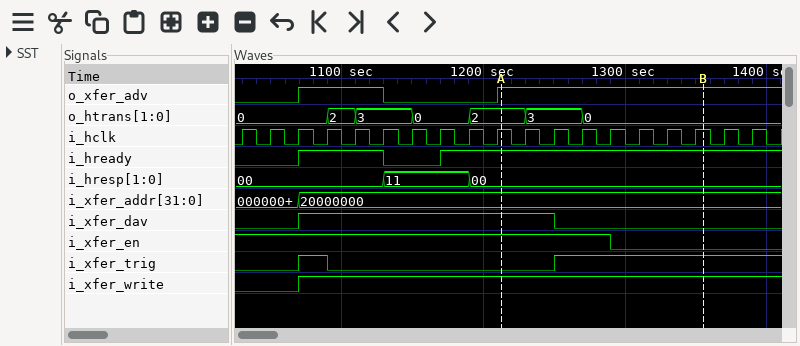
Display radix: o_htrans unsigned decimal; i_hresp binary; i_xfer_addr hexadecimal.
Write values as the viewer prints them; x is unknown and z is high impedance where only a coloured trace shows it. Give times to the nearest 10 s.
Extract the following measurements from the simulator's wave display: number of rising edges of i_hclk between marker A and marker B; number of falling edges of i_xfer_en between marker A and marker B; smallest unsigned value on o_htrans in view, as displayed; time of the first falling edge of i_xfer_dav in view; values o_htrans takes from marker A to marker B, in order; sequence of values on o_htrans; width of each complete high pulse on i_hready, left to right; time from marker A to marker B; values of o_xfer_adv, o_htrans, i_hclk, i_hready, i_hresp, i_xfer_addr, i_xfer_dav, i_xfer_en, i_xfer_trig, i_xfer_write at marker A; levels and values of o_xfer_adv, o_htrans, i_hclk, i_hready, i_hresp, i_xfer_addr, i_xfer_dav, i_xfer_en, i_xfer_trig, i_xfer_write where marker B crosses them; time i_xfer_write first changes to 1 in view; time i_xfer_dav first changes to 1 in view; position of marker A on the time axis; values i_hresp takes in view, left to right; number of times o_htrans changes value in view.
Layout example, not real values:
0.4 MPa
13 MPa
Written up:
7
1
0
1250 s
2, 3, 0
0, 2, 3, 0, 2, 3, 0
60 s
140 s
o_xfer_adv=1, o_htrans=2, i_hclk=1, i_hready=1, i_hresp=00, i_xfer_addr=20000000, i_xfer_dav=1, i_xfer_en=1, i_xfer_trig=0, i_xfer_write=1
o_xfer_adv=1, o_htrans=0, i_hclk=1, i_hready=1, i_hresp=00, i_xfer_addr=20000000, i_xfer_dav=0, i_xfer_en=0, i_xfer_trig=1, i_xfer_write=1
1070 s
1070 s
1210 s
00, 11, 00
6
